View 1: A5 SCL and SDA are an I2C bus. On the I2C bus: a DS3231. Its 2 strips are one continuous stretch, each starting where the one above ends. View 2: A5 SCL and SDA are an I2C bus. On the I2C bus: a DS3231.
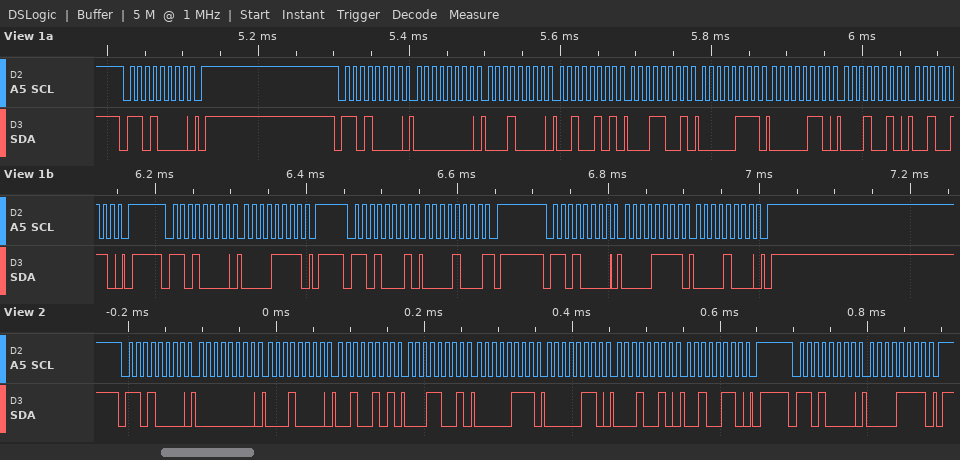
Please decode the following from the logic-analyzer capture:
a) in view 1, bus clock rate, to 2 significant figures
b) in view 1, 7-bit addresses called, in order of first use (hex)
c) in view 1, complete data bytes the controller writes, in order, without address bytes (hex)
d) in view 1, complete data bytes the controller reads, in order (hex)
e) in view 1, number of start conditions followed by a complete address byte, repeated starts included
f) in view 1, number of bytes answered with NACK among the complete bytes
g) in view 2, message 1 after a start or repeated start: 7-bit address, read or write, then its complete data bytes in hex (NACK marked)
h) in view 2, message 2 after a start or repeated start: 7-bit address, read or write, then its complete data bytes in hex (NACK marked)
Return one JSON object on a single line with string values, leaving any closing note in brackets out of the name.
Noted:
{"in view 1, bus clock rate, to 2 significant figures": "100 kHz", "in view 1, 7-bit addresses called, in order of first use": "0x68", "in view 1, complete data bytes the controller writes, in order, without address bytes": "00 10 25 19 07 06 12 26 0F 0F 08", "in view 1, complete data bytes the controller reads, in order": "08", "in view 1, number of start conditions followed by a complete address byte, repeated starts included": "5", "in view 1, number of bytes answered with NACK among the complete bytes": "1", "in view 2, message 1 after a start or repeated start: 7-bit address, read or write, then its complete data bytes in hex": "0x68 write: 00 10 25 19 07 06 12 26", "in view 2, message 2 after a start or repeated start: 7-bit address, read or write, then its complete data bytes in hex": "0x68 write: 0F"}
